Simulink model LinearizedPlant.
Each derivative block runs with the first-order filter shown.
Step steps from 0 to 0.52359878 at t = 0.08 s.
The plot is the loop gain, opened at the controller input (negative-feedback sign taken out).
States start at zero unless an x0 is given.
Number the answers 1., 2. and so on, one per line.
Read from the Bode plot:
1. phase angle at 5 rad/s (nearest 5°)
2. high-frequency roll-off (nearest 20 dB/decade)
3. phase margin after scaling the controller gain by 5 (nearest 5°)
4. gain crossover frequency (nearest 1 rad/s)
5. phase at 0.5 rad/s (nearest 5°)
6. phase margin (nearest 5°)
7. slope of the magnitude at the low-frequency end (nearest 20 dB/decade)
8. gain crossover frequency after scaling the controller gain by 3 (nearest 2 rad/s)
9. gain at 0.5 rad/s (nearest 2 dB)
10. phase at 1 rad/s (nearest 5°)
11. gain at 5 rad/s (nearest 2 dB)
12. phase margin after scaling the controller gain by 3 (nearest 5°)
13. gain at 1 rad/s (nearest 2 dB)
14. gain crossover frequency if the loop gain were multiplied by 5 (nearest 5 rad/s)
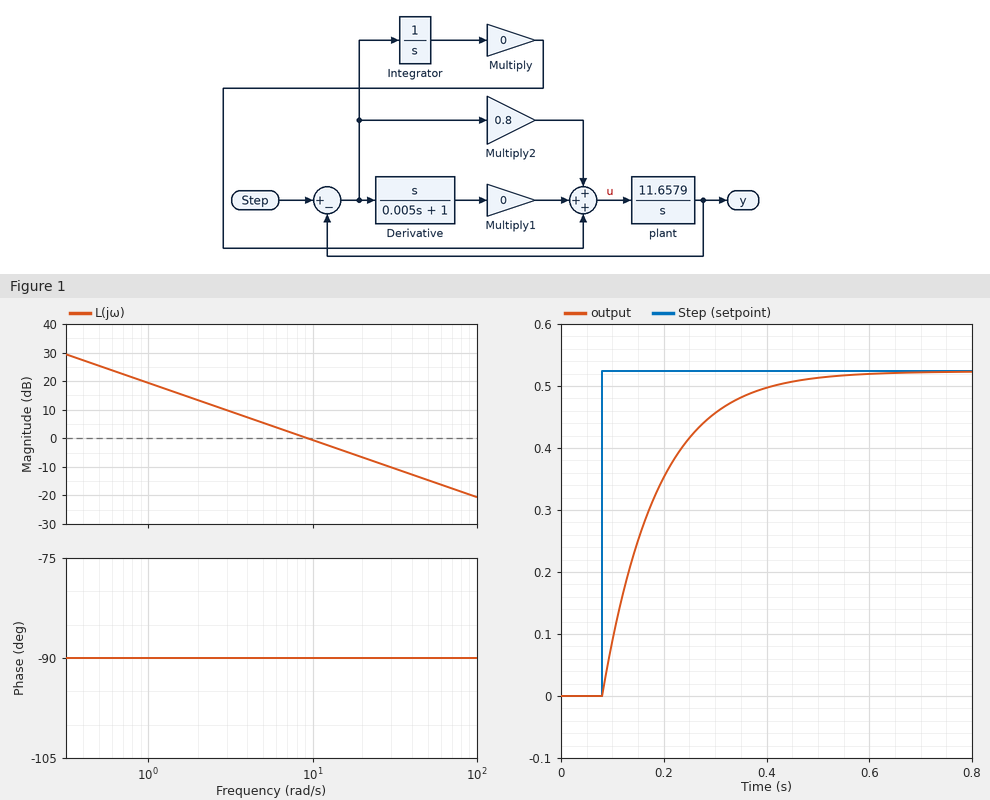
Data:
1. -90°
2. -20 dB/decade
3. 90°
4. 9 rad/s
5. -90°
6. 90°
7. -20 dB/decade
8. 28 rad/s
9. 26 dB
10. -90°
11. 6 dB
12. 90°
13. 20 dB
14. 45 rad/s
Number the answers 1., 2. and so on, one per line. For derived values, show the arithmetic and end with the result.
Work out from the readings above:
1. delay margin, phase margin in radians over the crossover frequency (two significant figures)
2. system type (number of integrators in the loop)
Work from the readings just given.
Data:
1. 90 × π / 180 / 9 = 0.17 s
2. 1
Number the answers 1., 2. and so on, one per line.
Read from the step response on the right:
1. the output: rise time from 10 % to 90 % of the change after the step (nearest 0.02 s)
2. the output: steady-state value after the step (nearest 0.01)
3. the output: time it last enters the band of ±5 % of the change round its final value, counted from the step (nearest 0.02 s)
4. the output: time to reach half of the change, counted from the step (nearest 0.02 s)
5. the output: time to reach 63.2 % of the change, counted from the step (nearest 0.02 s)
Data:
1. 0.24 s
2. 0.52
3. 0.32 s
4. 0.08 s
5. 0.10 s
